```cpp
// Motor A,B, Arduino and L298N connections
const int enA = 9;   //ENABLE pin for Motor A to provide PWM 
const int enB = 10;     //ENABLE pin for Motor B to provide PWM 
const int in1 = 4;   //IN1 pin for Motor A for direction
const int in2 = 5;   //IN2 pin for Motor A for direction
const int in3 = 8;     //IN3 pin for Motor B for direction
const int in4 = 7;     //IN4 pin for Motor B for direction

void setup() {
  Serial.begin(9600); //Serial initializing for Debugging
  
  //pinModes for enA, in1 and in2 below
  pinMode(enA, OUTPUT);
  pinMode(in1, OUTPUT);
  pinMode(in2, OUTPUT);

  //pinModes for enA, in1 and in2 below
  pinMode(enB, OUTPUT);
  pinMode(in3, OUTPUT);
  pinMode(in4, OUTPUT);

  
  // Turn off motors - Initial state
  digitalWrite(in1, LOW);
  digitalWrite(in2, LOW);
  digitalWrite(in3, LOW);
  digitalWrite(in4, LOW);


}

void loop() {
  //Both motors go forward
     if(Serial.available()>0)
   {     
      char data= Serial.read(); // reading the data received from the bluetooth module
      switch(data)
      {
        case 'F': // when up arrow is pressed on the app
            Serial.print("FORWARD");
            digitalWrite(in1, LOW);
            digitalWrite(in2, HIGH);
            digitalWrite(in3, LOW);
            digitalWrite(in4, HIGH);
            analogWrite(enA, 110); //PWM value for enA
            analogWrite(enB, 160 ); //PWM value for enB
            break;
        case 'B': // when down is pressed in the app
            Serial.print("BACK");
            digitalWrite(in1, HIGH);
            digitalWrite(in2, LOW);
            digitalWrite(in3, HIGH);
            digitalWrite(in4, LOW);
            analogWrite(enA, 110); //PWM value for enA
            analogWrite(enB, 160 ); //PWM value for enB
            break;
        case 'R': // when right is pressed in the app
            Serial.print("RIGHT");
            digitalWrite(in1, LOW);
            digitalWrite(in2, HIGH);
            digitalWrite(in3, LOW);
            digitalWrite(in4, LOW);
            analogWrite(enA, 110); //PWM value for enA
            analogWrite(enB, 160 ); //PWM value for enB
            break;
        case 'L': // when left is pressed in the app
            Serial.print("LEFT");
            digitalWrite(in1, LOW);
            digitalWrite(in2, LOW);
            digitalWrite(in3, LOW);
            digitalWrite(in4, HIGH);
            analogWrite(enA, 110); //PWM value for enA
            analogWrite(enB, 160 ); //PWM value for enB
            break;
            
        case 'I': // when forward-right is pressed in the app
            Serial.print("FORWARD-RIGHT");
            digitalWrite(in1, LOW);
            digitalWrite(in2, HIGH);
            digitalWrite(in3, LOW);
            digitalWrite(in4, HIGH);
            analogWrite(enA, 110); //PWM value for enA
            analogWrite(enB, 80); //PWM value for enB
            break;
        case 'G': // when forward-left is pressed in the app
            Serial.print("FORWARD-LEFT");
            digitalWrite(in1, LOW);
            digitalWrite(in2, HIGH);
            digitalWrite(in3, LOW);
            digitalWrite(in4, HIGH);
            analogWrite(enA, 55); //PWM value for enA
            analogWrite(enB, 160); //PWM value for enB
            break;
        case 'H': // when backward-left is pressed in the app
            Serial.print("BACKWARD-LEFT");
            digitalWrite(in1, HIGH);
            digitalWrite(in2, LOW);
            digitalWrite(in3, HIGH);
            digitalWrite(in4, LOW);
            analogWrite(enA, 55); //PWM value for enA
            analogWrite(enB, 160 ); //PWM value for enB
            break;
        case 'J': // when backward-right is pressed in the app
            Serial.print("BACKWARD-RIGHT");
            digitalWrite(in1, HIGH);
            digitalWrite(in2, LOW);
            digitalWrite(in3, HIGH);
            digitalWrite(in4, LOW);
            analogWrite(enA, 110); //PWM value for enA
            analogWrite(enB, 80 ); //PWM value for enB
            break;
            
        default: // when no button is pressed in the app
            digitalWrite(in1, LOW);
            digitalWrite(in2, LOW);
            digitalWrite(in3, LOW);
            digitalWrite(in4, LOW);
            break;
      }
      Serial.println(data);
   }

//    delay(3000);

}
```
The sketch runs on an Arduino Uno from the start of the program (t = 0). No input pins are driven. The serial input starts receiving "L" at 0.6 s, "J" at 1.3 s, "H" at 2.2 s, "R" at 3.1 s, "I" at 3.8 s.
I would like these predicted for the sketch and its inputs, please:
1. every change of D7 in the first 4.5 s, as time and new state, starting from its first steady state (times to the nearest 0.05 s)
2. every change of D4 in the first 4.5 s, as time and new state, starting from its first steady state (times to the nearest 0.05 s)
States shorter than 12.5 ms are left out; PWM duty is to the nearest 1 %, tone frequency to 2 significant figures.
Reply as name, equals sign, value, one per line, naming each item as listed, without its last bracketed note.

every change of D7 in the first 4.5 s, as time and new state, starting from its first steady state = 0 s low; 0.6 s high; 1.3 s low; 3.8 s high
every change of D4 in the first 4.5 s, as time and new state, starting from its first steady state = 0 s low; 1.3 s high; 3.1 s low
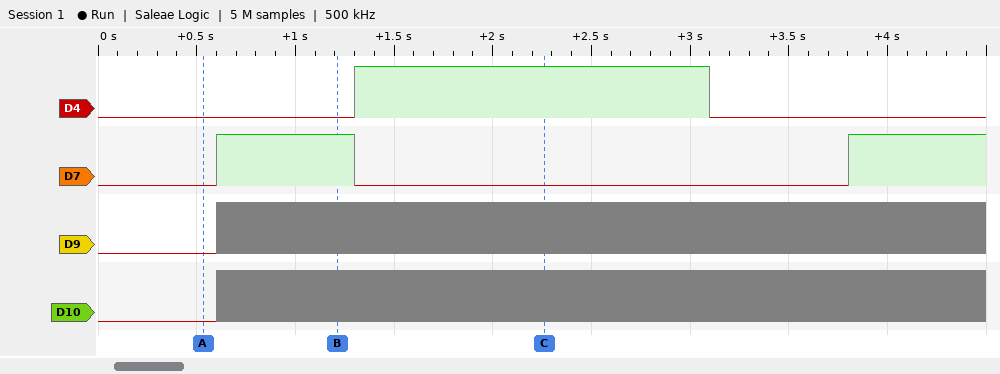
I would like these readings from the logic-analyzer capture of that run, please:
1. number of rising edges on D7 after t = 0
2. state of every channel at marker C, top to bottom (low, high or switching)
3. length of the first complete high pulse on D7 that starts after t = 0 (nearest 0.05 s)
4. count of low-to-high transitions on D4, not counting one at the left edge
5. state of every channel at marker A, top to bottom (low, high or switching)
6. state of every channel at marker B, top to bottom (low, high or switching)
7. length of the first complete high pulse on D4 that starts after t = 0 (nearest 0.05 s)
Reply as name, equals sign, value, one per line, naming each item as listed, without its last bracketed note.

number of rising edges on D7 after t = 0 = 2
state of every channel at marker C, top to bottom = D4 high, D7 low, D9 switching, D10 switching
length of the first complete high pulse on D7 that starts after t = 0 = 0.70 s
count of low-to-high transitions on D4, not counting one at the left edge = 1
state of every channel at marker A, top to bottom = D4 low, D7 low, D9 low, D10 low
state of every channel at marker B, top to bottom = D4 low, D7 high, D9 switching, D10 switching
length of the first complete high pulse on D4 that starts after t = 0 = 1.80 s
